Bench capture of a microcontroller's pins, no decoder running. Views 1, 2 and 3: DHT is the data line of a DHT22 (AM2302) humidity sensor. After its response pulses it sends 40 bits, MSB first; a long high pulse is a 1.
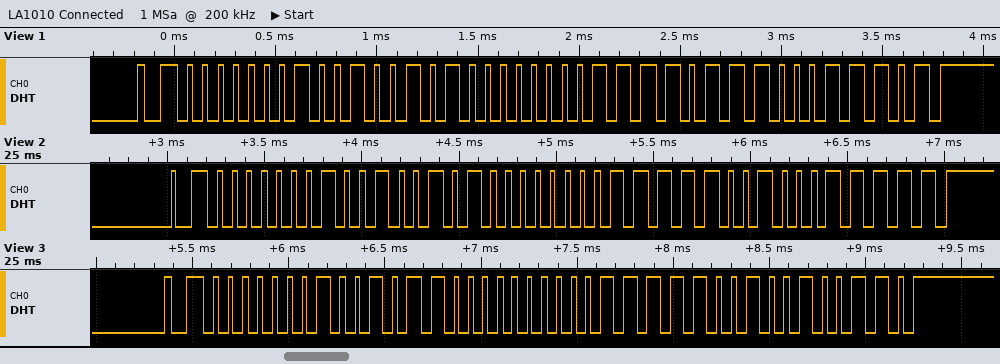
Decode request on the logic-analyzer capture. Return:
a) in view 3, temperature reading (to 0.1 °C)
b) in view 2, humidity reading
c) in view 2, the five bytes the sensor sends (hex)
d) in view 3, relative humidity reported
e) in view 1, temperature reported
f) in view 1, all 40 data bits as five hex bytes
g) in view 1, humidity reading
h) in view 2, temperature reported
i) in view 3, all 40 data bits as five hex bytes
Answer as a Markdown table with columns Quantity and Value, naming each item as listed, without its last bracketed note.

| Quantity | Value |
|---|---|
| in view 3, temperature reading | 24.9 °C |
| in view 2, humidity reading | 29.3 % |
| in view 2, the five bytes the sensor sends | 01 25 00 F9 1F |
| in view 3, relative humidity reported | 30.0 % |
| in view 1, temperature reported | 24.7 °C |
| in view 1, all 40 data bits as five hex bytes | 01 25 00 F7 1D |
| in view 1, humidity reading | 29.3 % |
| in view 2, temperature reported | 24.9 °C |
| in view 3, all 40 data bits as five hex bytes | 01 2C 00 F9 26 |
